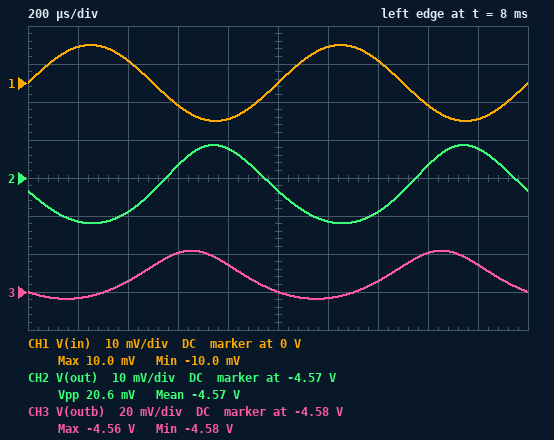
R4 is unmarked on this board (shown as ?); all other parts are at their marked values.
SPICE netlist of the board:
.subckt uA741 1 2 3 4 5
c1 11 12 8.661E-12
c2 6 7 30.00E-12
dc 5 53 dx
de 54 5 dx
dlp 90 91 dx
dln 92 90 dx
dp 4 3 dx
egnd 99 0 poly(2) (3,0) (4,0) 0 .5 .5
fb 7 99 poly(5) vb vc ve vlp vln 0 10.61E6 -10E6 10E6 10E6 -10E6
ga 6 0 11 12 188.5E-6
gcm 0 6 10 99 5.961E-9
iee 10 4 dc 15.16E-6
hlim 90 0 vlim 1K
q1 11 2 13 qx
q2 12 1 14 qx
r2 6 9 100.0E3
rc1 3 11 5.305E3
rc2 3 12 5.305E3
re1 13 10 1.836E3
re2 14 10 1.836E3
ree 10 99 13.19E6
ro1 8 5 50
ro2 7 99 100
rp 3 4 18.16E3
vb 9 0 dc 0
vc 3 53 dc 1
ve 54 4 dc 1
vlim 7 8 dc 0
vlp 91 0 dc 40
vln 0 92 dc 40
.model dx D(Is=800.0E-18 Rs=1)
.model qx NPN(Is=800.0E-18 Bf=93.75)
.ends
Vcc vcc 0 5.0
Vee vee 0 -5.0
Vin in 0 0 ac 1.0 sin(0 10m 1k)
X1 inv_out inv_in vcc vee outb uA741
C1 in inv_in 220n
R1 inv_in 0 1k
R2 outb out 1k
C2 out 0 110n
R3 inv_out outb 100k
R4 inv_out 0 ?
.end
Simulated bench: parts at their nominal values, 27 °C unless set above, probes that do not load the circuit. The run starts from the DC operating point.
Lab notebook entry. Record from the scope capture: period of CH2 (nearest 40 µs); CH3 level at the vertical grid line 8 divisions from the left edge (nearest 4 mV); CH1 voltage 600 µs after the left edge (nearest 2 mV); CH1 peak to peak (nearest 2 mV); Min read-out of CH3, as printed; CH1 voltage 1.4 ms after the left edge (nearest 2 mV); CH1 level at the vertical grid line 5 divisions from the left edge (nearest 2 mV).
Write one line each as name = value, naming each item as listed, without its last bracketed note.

period of CH2 = 1.00 ms
CH3 level at the vertical grid line 8 divisions from the left edge = -4.560 V
CH1 voltage 600 µs after the left edge = -6 mV
CH1 peak to peak = 20 mV
Min read-out of CH3, as printed = -4.58 V
CH1 voltage 1.4 ms after the left edge = 6 mV
CH1 level at the vertical grid line 5 divisions from the left edge = 0 V
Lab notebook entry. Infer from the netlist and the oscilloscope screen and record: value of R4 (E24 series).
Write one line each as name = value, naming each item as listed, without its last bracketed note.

value of R4 = 390 Ω
